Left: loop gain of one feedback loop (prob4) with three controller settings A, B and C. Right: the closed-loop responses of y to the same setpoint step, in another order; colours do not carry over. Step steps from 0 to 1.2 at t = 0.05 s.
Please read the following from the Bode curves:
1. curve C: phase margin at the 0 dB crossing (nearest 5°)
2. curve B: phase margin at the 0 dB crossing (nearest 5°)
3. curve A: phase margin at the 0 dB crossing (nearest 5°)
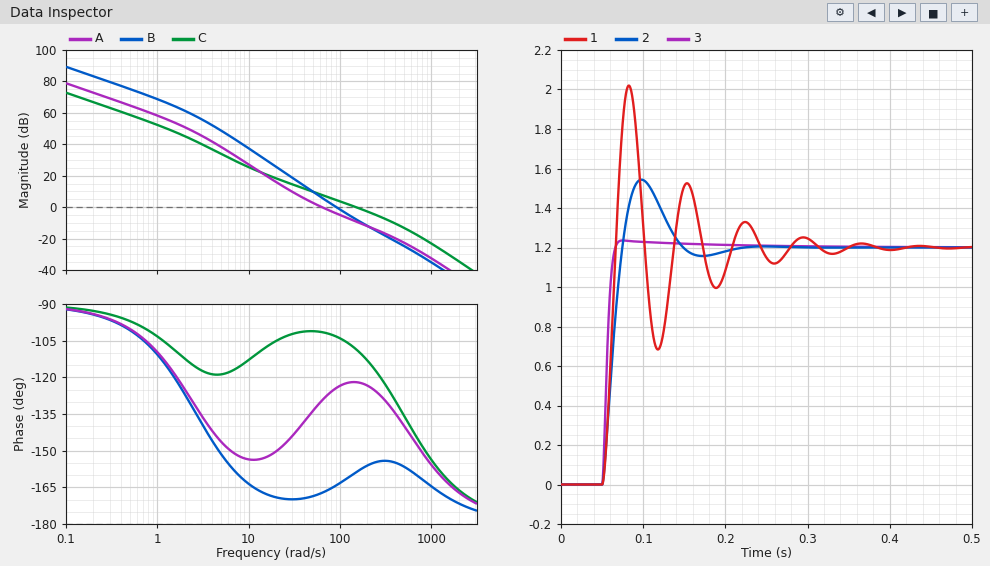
70°
15°
50°
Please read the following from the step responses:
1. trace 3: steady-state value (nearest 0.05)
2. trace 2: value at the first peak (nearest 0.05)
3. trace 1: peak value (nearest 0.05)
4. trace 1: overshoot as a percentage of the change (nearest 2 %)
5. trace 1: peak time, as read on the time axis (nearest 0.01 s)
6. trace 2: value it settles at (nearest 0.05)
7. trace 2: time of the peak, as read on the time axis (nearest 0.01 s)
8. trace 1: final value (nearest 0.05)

1.20
1.55
2.00
68 %
0.08 s
1.20
0.10 s
1.20
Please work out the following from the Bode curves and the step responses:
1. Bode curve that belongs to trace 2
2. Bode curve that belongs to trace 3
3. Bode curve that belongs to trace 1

A
C
B
